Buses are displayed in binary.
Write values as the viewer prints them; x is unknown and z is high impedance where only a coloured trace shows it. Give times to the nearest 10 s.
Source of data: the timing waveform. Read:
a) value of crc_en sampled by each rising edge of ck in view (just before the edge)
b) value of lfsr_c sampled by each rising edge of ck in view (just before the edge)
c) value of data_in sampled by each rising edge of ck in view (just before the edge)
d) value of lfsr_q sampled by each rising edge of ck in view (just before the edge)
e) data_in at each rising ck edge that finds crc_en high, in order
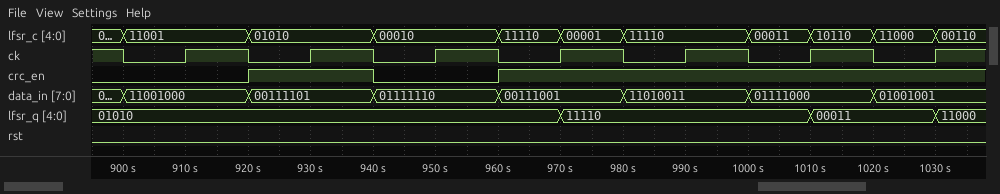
0 1 0 1 1 1 1
11001, 01010, 00010, 11110, 11110, 00011, 11000
11001000, 00111101, 01111110, 00111001, 11010011, 01111000, 01001001
01010, 01010, 01010, 01010, 11110, 11110, 00011
00111101, 00111001, 11010011, 01111000, 01001001
